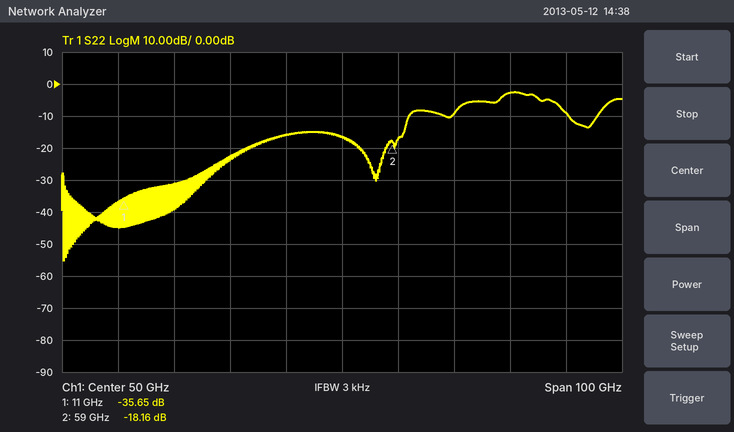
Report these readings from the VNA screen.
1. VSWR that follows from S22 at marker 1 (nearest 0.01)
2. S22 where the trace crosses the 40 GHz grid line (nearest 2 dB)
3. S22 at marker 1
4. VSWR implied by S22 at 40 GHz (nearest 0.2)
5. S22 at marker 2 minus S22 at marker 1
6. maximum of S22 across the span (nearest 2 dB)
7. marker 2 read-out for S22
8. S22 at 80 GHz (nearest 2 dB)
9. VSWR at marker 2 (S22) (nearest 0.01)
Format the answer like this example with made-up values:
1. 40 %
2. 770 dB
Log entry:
1. 1.03
2. -16 dB
3. -35.65 dB
4. 1.4
5. 17.49 dB
6. -2 dB
7. -18.16 dB
8. -2 dB
9. 1.28
